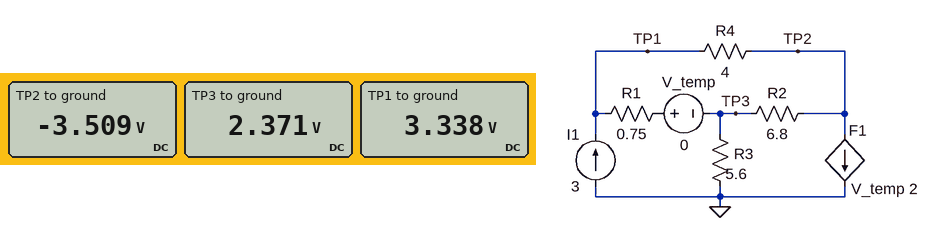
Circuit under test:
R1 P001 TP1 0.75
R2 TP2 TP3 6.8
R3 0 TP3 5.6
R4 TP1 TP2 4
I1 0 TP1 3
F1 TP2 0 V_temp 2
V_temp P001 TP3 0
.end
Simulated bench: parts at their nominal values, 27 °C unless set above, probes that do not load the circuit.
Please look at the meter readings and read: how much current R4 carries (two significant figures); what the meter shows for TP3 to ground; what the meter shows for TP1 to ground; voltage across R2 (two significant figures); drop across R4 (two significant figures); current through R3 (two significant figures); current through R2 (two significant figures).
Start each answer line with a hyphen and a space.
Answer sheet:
- 1.7 A
- 2.371 V
- 3.338 V
- 5.9 V
- 6.8 V
- 420 mA
- 860 mA
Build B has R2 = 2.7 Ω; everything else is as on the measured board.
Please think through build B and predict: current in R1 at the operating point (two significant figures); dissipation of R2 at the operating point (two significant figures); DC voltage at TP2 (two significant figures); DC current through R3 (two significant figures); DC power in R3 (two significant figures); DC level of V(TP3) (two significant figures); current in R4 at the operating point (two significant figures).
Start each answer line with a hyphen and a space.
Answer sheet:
- 1.6 A
- 7.7 W
- -5.3 V
- 130 mA
- 92 mW
- -720 mV
- 1.4 A
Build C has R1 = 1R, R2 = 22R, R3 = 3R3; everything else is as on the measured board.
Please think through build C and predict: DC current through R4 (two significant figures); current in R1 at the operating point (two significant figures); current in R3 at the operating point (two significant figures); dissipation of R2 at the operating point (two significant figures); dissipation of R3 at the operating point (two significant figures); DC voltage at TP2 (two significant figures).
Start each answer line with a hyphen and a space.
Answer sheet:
- 1.9 A
- 1.1 A
- 800 mA
- 1.9 W
- 2.1 W
- -3.9 V
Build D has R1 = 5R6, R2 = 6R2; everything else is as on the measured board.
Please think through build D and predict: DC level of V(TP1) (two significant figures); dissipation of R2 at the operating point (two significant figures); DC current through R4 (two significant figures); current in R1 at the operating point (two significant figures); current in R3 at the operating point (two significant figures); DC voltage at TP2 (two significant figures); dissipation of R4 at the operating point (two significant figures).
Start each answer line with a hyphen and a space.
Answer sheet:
- 11 V
- 400 mW
- 1.9 A
- 1.1 A
- 830 mA
- 3.1 V
- 15 W
